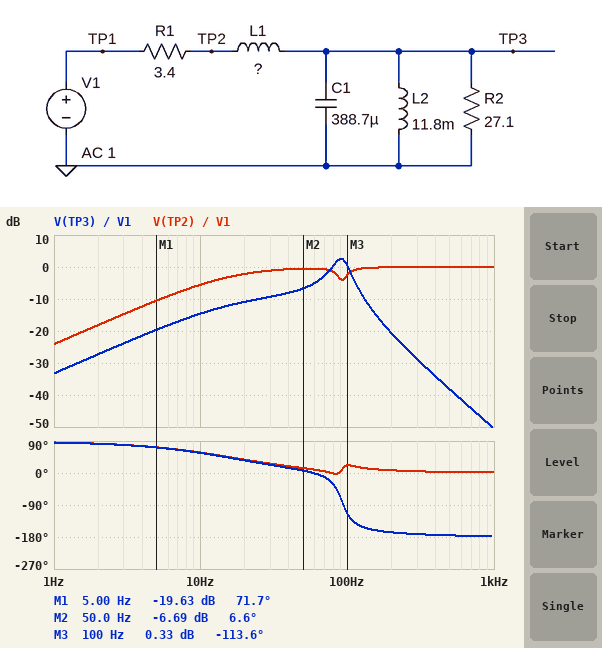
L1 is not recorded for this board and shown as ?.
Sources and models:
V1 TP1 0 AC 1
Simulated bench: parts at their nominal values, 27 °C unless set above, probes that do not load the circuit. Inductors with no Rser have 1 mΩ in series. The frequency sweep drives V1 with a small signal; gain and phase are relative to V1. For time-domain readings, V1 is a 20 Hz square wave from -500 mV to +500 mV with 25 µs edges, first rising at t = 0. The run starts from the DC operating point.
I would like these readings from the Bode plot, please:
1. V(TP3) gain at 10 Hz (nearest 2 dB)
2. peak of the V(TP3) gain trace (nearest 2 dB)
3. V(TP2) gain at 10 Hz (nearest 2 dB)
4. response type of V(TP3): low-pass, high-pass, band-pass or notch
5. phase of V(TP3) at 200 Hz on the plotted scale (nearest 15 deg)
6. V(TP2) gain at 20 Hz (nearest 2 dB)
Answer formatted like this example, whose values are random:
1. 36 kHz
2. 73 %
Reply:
1. -14 dB
2. 2 dB
3. -6 dB
4. band-pass
5. -165 deg
6. -2 dB
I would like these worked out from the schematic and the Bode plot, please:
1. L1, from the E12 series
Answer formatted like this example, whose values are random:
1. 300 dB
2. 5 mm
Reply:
1. 22 mH
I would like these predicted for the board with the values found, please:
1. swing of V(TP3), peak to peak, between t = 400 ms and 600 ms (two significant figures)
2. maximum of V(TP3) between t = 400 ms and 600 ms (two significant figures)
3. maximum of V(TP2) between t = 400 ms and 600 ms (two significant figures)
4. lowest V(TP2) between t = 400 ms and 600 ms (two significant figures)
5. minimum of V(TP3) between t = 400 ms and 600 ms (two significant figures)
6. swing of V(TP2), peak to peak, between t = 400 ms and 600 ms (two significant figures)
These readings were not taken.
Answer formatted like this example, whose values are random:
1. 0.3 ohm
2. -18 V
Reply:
1. 860 mV
2. 430 mV
3. 940 mV
4. -940 mV
5. -430 mV
6. 1.9 V
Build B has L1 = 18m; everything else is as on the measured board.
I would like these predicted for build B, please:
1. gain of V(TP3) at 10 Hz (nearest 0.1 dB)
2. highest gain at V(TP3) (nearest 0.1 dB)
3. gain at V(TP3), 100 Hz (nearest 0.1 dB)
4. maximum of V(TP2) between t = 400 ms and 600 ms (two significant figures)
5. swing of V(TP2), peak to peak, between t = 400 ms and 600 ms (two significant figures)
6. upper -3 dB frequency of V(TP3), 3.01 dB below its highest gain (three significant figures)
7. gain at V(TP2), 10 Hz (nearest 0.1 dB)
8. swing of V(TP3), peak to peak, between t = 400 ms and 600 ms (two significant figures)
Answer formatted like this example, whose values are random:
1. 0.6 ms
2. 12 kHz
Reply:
1. -14.3 dB
2. 2.9 dB
3. 2.0 dB
4. 950 mV
5. 1.9 V
6. 106 Hz
7. -6.3 dB
8. 990 mV
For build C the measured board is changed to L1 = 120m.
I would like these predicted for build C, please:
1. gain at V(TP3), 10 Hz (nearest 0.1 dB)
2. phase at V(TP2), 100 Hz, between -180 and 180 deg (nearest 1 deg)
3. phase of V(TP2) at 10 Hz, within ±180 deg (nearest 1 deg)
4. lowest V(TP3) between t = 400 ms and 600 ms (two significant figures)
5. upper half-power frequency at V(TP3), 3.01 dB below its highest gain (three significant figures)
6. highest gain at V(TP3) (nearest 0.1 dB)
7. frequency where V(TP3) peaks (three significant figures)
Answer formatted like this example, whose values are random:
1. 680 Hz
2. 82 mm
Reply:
1. -21.5 dB
2. 3 deg
3. 22 deg
4. -100 mV
5. 84.6 Hz
6. -6.9 dB
7. 77.1 Hz
